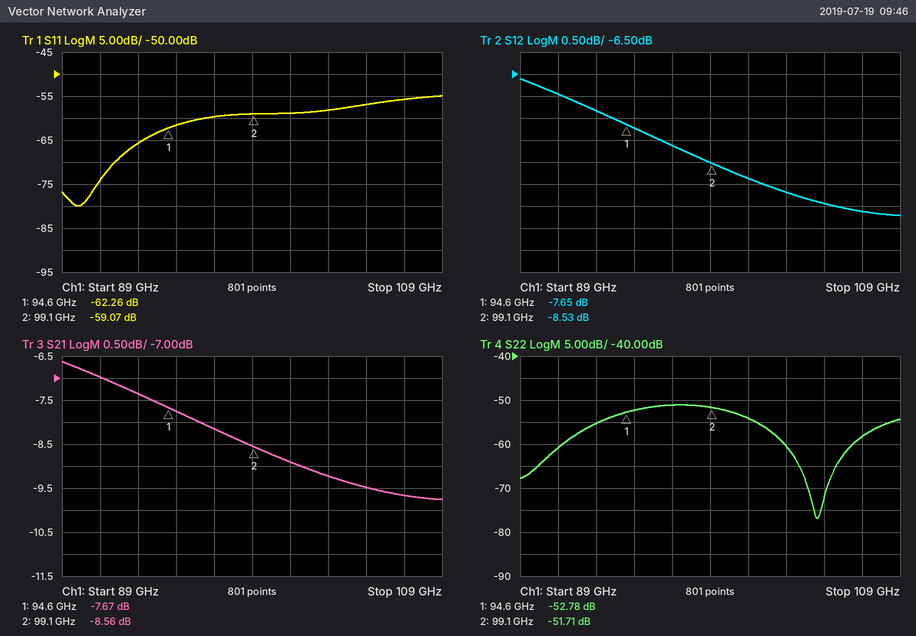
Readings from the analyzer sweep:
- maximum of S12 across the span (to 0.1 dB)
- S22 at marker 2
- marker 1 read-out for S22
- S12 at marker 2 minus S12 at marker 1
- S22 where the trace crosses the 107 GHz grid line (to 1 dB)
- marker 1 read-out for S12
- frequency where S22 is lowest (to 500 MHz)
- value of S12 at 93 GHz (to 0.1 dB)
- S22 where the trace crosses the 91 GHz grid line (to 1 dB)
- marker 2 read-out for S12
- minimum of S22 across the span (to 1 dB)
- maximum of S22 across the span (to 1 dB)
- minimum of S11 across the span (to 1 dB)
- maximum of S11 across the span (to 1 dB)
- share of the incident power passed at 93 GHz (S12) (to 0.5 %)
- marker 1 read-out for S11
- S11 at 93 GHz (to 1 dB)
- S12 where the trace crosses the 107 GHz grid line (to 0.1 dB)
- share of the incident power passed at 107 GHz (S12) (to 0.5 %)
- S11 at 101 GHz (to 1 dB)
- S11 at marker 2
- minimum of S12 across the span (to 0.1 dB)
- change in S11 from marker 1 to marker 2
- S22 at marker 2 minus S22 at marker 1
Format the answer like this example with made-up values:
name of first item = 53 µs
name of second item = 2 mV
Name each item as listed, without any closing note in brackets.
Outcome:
maximum of S12 across the span = -6.6 dB
S22 at marker 2 = -51.71 dB
marker 1 read-out for S22 = -52.78 dB
S12 at marker 2 minus S12 at marker 1 = -0.88 dB
S22 where the trace crosses the 107 GHz grid line = -58 dB
marker 1 read-out for S12 = -7.65 dB
frequency where S22 is lowest = 104.5 GHz
value of S12 at 93 GHz = -7.3 dB
S22 where the trace crosses the 91 GHz grid line = -61 dB
marker 2 read-out for S12 = -8.53 dB
minimum of S22 across the span = -77 dB
maximum of S22 across the span = -51 dB
minimum of S11 across the span = -80 dB
maximum of S11 across the span = -55 dB
share of the incident power passed at 93 GHz (S12) = 18.5 %
marker 1 read-out for S11 = -62.26 dB
S11 at 93 GHz = -66 dB
S12 where the trace crosses the 107 GHz grid line = -9.6 dB
share of the incident power passed at 107 GHz (S12) = 11.0 %
S11 at 101 GHz = -59 dB
S11 at marker 2 = -59.07 dB
minimum of S12 across the span = -9.7 dB
change in S11 from marker 1 to marker 2 = 3.19 dB
S22 at marker 2 minus S22 at marker 1 = 1.07 dB
